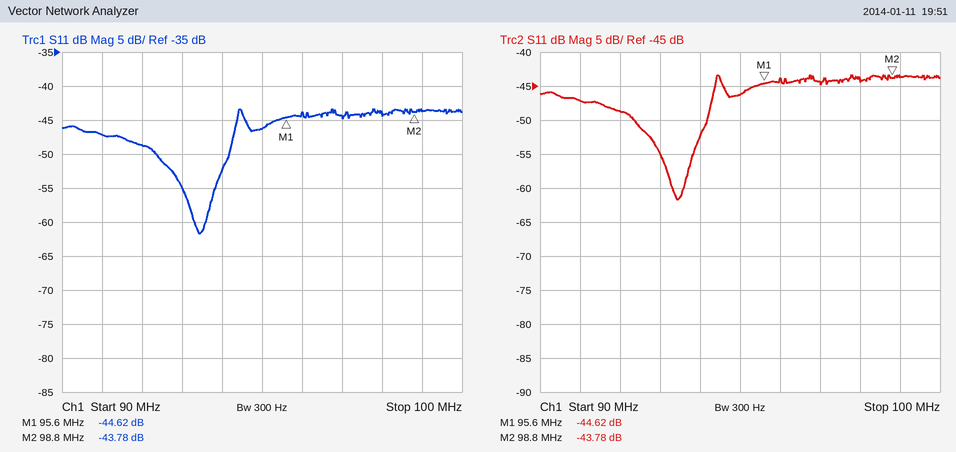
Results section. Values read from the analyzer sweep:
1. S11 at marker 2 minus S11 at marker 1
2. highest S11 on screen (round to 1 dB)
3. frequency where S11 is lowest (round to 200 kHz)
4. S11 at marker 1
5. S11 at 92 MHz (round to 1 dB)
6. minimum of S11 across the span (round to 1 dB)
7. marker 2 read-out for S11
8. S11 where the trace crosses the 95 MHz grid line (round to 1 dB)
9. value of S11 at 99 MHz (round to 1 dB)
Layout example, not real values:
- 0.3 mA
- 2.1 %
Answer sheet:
- 0.84 dB
- -43 dB
- 93.4 MHz
- -44.62 dB
- -49 dB
- -62 dB
- -43.78 dB
- -46 dB
- -44 dB
